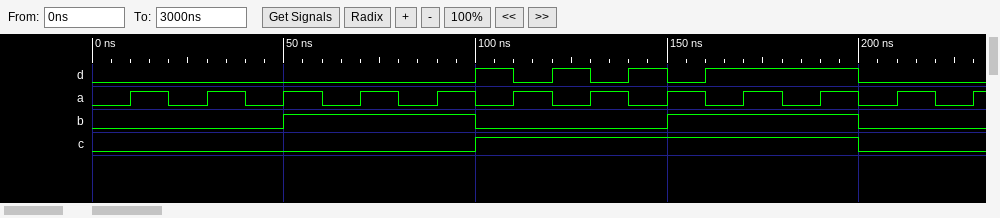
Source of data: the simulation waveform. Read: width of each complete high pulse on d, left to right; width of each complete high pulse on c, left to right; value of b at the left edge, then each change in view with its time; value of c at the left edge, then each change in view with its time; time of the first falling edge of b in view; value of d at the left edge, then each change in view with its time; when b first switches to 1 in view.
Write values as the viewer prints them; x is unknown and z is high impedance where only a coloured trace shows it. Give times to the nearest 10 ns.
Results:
10 ns, 10 ns, 10 ns, 40 ns
100 ns
0, 1 at 50 ns, 0 at 100 ns, 1 at 150 ns, 0 at 200 ns
0, 1 at 100 ns, 0 at 200 ns
100 ns
0, 1 at 100 ns, 0 at 110 ns, 1 at 120 ns, 0 at 130 ns, 1 at 140 ns, 0 at 150 ns, 1 at 160 ns, 0 at 200 ns
50 ns
